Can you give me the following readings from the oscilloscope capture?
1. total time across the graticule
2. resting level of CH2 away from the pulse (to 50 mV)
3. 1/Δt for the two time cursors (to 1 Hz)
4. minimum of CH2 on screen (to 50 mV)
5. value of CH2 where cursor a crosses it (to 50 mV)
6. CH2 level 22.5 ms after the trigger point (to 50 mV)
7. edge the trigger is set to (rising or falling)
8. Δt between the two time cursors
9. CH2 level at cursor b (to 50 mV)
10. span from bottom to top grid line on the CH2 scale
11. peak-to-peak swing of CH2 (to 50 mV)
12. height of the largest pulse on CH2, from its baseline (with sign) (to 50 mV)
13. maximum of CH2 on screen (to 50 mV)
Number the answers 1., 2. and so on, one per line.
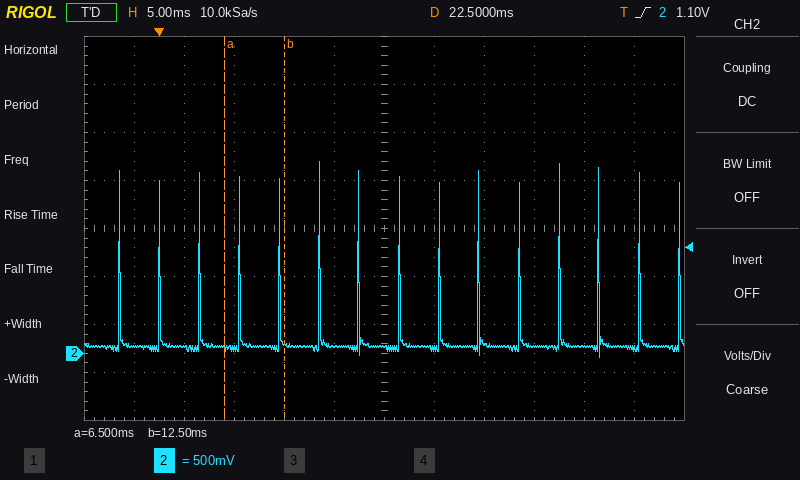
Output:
1. 60 ms
2. 50 mV
3. 167 Hz
4. -50 mV
5. 50 mV
6. 50 mV
7. rising
8. 6.0 ms
9. 100 mV
10. 4 V
11. 2.05 V
12. +1.95 V
13. 2.00 V
